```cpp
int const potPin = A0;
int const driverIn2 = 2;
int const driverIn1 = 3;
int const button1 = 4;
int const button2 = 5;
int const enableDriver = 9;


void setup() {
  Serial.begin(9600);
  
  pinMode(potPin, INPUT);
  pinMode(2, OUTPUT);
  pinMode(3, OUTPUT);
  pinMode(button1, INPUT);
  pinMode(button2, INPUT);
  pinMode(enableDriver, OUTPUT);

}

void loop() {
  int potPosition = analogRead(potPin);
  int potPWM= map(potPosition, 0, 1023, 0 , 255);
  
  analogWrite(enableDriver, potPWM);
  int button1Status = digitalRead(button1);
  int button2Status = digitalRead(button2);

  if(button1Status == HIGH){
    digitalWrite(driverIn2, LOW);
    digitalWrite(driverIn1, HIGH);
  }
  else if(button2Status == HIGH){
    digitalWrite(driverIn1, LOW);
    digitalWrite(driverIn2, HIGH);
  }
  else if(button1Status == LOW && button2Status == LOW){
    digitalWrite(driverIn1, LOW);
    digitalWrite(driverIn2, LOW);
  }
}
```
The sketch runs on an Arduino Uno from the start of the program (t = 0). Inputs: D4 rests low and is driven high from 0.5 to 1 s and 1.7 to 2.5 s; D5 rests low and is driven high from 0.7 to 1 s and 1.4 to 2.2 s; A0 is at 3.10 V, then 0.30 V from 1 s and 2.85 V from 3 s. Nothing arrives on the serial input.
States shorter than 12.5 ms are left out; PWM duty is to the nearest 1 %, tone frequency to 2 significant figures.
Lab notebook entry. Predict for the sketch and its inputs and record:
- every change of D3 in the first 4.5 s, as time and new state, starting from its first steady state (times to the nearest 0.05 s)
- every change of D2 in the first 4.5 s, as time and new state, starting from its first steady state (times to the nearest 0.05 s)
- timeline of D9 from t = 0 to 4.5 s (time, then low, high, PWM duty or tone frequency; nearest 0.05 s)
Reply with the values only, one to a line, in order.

0 s low; 0.5 s high; 1 s low; 1.7 s high; 2.5 s low
0 s low; 1.4 s high; 1.7 s low
0 s PWM 62 %; 1 s PWM 6 %; 3 s PWM 57 %
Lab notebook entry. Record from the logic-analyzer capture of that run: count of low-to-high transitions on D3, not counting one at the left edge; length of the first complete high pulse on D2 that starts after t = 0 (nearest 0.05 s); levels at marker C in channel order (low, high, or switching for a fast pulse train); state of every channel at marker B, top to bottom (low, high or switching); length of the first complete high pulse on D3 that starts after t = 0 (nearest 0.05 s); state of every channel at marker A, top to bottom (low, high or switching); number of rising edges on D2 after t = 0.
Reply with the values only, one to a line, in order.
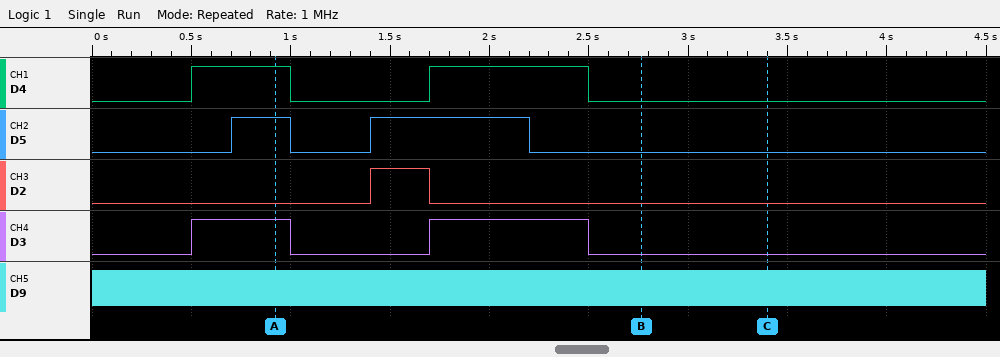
2
0.30 s
D4 low, D5 low, D2 low, D3 low, D9 switching
D4 low, D5 low, D2 low, D3 low, D9 switching
0.50 s
D4 high, D5 high, D2 low, D3 high, D9 switching
1
